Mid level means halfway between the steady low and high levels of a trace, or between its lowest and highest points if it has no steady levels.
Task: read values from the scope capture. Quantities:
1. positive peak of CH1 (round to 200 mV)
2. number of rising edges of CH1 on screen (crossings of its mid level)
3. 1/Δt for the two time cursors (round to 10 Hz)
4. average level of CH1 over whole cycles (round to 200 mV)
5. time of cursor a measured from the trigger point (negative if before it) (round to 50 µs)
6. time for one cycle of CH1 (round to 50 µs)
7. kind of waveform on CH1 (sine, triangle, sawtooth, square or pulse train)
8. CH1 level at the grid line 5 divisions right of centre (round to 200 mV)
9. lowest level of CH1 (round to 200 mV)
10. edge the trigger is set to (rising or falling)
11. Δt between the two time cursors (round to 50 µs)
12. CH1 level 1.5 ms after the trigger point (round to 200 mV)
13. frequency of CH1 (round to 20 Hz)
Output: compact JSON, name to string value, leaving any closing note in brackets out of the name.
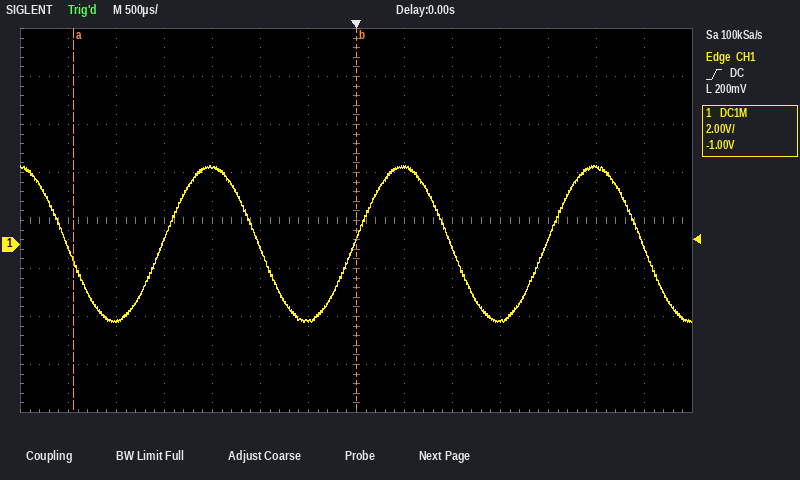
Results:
{"positive peak of CH1": "3.2 V", "number of rising edges of CH1 on screen": "3", "1/Δt for the two time cursors": "340 Hz", "average level of CH1 over whole cycles": "0.0 V", "time of cursor a measured from the trigger point (negative if before it)": "-2.95 ms", "time for one cycle of CH1": "2.00 ms", "kind of waveform on CH1": "sine", "CH1 level at the grid line 5 divisions right of centre": "3.2 V", "lowest level of CH1": "-3.2 V", "edge the trigger is set to": "rising", "Δt between the two time cursors": "2.95 ms", "CH1 level 1.5 ms after the trigger point": "-3.2 V", "frequency of CH1": "500 Hz"}
